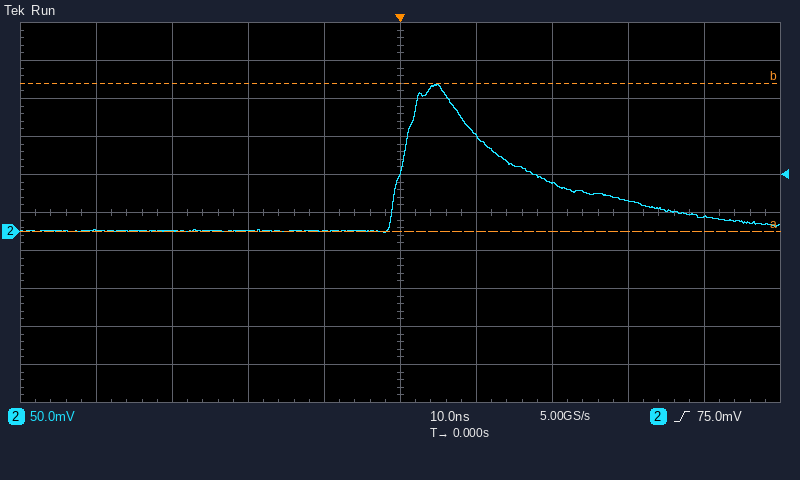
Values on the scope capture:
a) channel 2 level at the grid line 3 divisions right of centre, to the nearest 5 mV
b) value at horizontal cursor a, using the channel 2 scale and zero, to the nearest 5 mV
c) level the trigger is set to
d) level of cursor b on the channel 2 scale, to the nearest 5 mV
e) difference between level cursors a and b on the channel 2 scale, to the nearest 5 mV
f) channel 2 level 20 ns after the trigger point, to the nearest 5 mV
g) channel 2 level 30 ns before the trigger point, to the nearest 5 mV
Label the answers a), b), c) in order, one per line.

a) 40 mV
b) 0 mV
c) 75.0 mV
d) 195 mV
e) 195 mV
f) 65 mV
g) 0 mV
